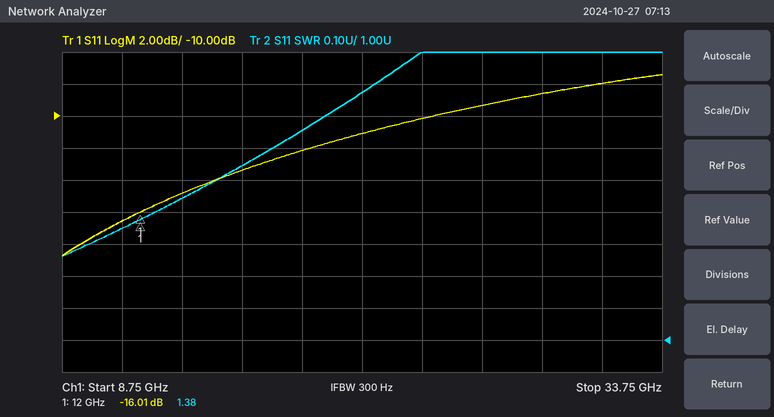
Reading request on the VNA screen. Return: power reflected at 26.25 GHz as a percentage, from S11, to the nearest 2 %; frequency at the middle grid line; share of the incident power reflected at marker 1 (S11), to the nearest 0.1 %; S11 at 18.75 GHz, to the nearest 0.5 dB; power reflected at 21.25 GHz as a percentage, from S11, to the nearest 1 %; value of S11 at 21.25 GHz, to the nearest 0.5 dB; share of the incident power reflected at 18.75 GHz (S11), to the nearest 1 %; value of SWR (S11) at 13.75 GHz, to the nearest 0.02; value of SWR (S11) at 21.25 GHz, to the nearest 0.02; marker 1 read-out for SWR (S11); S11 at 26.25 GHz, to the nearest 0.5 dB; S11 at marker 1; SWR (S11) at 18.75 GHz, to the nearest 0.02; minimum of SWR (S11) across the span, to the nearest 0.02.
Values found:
12 %
21.25 GHz
2.5 %
-12.0 dB
8 %
-11.0 dB
6 %
1.44
1.78
1.38
-9.5 dB
-16.01 dB
1.66
1.26
